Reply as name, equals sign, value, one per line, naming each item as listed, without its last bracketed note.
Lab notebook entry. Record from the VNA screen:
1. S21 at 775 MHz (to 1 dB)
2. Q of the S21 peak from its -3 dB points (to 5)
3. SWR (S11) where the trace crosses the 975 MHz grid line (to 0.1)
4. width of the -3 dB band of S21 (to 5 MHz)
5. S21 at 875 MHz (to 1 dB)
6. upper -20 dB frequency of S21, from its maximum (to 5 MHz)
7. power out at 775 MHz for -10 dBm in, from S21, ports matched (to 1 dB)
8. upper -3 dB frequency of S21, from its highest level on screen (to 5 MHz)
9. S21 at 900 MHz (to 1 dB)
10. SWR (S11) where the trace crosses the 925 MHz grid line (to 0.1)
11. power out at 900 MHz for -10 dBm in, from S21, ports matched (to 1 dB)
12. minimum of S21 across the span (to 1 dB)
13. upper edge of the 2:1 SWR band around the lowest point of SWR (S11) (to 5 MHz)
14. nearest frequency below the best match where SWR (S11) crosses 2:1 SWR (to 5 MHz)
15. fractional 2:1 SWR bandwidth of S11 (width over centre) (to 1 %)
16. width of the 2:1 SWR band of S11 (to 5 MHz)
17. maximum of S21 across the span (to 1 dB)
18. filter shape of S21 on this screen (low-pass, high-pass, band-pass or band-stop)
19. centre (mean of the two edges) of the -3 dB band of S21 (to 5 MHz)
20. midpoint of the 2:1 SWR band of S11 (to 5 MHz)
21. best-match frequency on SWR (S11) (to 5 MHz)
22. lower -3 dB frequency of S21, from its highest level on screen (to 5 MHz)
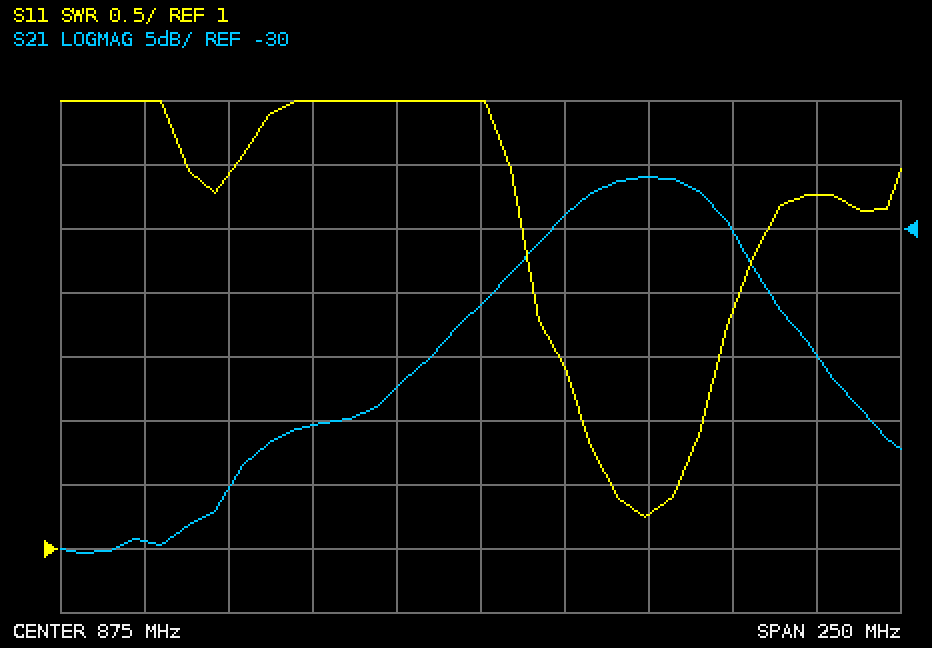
S21 at 775 MHz = -54 dB
Q of the S21 peak from its -3 dB points = 20
SWR (S11) where the trace crosses the 975 MHz grid line = 3.8
width of the -3 dB band of S21 = 45 MHz
S21 at 875 MHz = -36 dB
upper -20 dB frequency of S21, from its maximum = 995 MHz
power out at 775 MHz for -10 dBm in, from S21, ports matched = -64 dBm
upper -3 dB frequency of S21, from its highest level on screen = 945 MHz
S21 at 900 MHz = -29 dB
SWR (S11) where the trace crosses the 925 MHz grid line = 1.3
power out at 900 MHz for -10 dBm in, from S21, ports matched = -39 dBm
minimum of S21 across the span = -55 dB
upper edge of the 2:1 SWR band around the lowest point of SWR (S11) = 940 MHz
nearest frequency below the best match where SWR (S11) crosses 2:1 SWR = 905 MHz
fractional 2:1 SWR bandwidth of S11 (width over centre) = 4 %
width of the 2:1 SWR band of S11 = 35 MHz
maximum of S21 across the span = -26 dB
filter shape of S21 on this screen = band-pass
centre (mean of the two edges) of the -3 dB band of S21 = 925 MHz
midpoint of the 2:1 SWR band of S11 = 925 MHz
best-match frequency on SWR (S11) = 925 MHz
lower -3 dB frequency of S21, from its highest level on screen = 900 MHz
